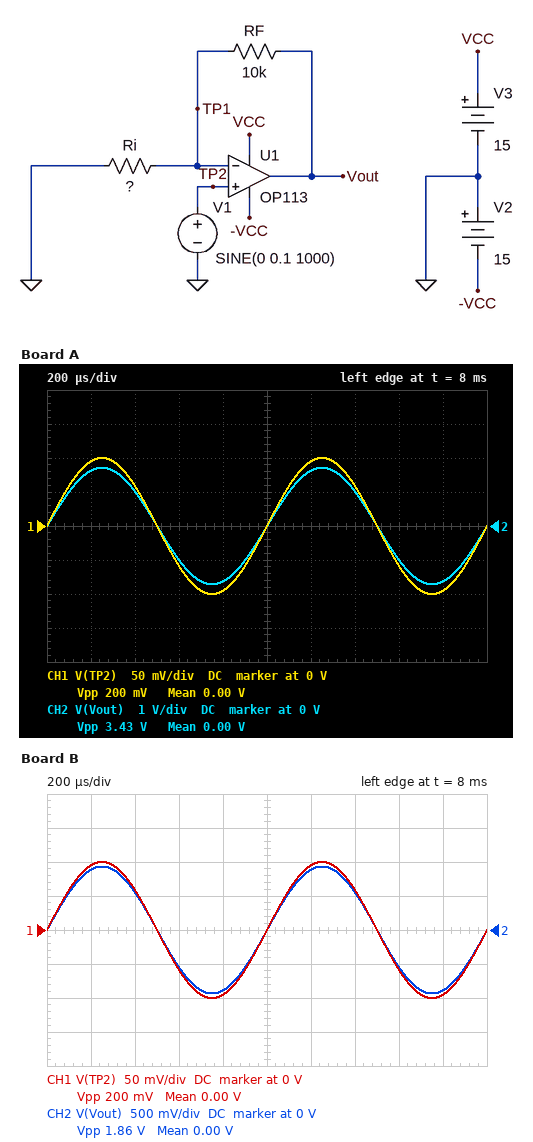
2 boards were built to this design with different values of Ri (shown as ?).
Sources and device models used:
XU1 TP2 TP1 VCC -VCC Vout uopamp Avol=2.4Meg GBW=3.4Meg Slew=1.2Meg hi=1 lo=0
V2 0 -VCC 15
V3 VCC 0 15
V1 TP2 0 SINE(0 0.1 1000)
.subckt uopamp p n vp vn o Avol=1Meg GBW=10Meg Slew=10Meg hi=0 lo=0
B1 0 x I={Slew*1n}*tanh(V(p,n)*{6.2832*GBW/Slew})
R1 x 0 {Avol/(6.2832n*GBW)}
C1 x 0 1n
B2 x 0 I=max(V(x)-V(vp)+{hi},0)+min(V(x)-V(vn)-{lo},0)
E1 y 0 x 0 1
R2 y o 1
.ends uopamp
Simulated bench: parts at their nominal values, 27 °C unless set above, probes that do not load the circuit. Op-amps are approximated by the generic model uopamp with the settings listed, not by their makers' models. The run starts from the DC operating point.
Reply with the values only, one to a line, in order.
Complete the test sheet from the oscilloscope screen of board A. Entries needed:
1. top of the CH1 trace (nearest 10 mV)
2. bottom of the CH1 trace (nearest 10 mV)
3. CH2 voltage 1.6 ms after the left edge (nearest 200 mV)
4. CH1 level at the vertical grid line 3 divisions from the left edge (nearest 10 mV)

100 mV
-100 mV
-1.0 V
-60 mV
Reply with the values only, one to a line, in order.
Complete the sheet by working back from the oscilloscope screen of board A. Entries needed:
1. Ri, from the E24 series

620 Ω
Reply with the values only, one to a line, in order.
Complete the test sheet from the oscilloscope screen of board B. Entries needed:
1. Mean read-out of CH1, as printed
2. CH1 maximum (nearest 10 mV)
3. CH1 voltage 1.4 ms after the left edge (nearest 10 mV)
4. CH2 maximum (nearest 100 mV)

0.00 V
100 mV
60 mV
900 mV
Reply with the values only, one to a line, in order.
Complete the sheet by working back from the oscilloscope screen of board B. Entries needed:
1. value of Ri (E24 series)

1.2 kΩ
